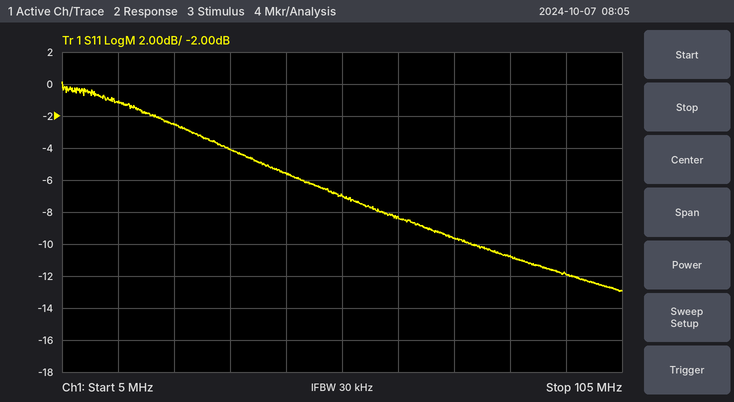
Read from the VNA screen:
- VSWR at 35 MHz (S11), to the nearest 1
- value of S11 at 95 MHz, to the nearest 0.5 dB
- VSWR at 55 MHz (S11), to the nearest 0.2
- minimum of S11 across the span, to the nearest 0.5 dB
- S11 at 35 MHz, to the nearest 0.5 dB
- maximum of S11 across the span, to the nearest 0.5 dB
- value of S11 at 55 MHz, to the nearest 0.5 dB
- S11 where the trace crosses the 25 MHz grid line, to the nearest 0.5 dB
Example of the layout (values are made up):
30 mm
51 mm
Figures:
4
-12.0 dB
2.6
-13.0 dB
-4.0 dB
0.0 dB
-7.0 dB
-2.5 dB
